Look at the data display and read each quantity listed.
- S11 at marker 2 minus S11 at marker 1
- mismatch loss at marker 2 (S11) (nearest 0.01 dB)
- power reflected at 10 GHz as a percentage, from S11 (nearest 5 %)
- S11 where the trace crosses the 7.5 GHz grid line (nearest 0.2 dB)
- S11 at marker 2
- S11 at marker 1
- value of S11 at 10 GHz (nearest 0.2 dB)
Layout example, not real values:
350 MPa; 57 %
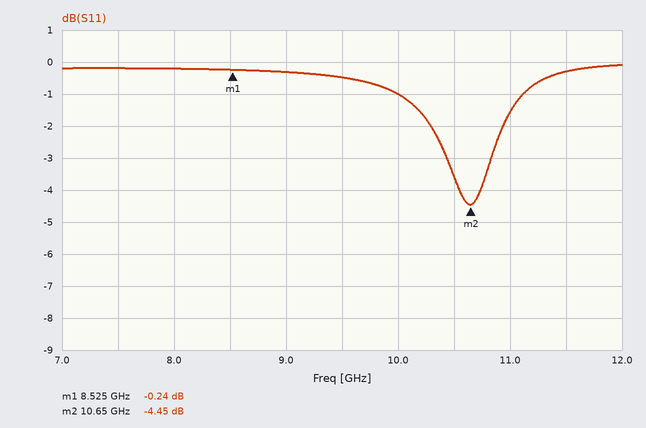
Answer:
-4.21 dB; 1.93 dB; 80 %; -0.2 dB; -4.45 dB; -0.24 dB; -1.0 dB
